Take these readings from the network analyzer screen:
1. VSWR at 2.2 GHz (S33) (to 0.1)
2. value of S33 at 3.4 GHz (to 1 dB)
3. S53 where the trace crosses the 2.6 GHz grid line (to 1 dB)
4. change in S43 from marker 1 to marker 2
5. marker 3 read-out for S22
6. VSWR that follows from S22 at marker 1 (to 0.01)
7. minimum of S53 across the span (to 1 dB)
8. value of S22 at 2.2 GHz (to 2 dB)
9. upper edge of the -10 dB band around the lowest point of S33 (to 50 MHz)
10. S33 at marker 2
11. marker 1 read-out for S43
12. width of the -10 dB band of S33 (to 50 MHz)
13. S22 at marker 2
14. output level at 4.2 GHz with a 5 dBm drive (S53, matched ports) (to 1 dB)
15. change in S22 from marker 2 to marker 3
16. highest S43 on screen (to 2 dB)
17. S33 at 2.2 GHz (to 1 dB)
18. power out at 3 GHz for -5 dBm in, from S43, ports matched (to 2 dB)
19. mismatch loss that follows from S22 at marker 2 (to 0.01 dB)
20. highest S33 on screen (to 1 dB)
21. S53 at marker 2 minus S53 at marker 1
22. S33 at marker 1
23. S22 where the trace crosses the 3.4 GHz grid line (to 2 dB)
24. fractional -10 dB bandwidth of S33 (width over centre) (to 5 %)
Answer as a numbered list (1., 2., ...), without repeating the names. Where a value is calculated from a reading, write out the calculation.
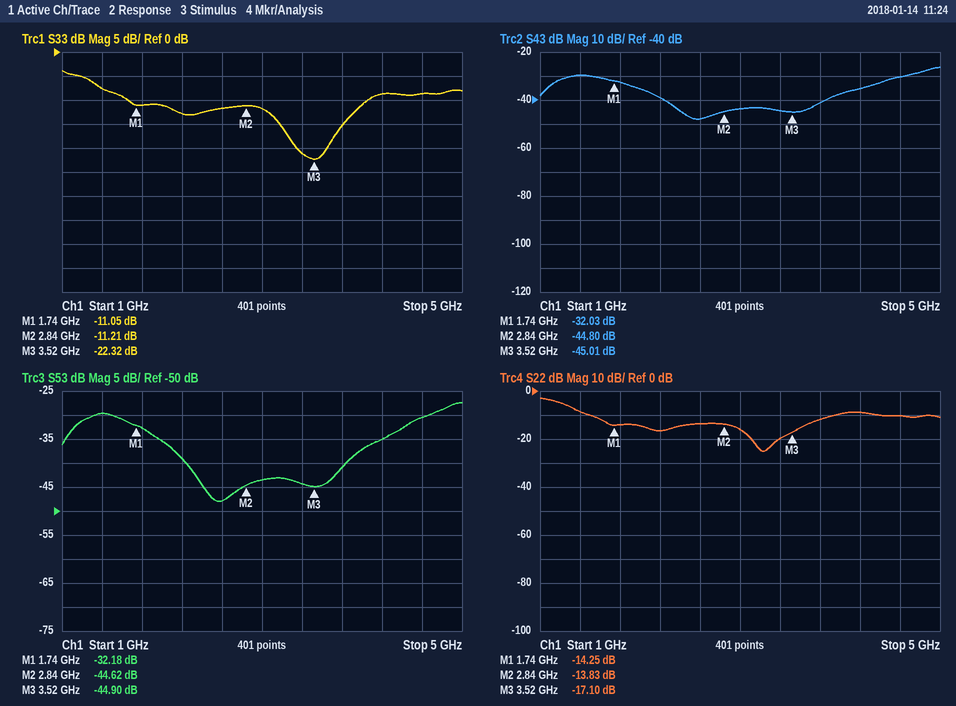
1. |Γ| = 10^(-13/20) = 0.2239; VSWR = (1 + 0.2239)/(1 − 0.2239) ≈ 1.6
2. -21 dB
3. -48 dB
4. -44.8 − (-32.03) = -12.77 dB
5. -17.10 dB
6. (1 + 0.1939)/(1 − 0.1939) ≈ 1.48
7. -48 dB
8. -16 dB
9. 4.05 GHz
10. -11.21 dB
11. -32.03 dB
12. 4.05 GHz − 1.65 GHz = 2.40 GHz
13. -13.83 dB
14. 5 dBm + (-35 dB) = -30 dBm
15. -17.1 − (-13.83) = -3.27 dB
16. -26 dB
17. -13 dB
18. -5 dBm + (-44 dB) = -48 dBm
19. −10 log10(1 − 10^(-13.83/10)) ≈ 0.18 dB
20. -4 dB
21. -44.62 − (-32.18) = -12.44 dB
22. -11.05 dB
23. -20 dB
24. 2.4 GHz / 2.85 GHz ≈ 84.2 %, so 85 % to the nearest 5 %
